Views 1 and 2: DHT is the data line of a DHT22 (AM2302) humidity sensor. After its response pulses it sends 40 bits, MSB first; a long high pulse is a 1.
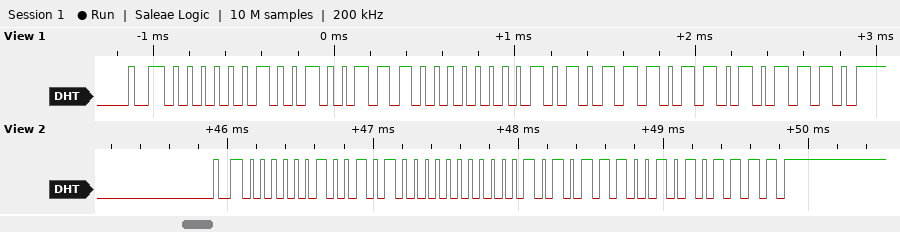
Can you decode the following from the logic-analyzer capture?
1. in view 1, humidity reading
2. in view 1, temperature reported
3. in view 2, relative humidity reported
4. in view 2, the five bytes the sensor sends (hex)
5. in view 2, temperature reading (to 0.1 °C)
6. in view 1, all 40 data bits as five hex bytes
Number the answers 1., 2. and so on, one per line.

1. 59.0 %
2. 34.9 °C
3. 59.2 %
4. 02 50 01 5C AF
5. 34.8 °C
6. 02 4E 01 5D AE
